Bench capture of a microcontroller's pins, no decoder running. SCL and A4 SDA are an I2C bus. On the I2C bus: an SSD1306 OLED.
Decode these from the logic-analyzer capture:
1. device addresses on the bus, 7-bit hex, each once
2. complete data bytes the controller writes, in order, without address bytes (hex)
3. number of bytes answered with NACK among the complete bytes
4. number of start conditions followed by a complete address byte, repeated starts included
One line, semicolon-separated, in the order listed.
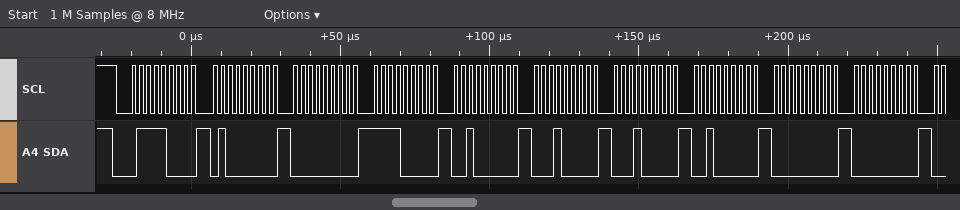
0x3C; 40 00 F0 20 10 10 20 00 00; 0; 1
